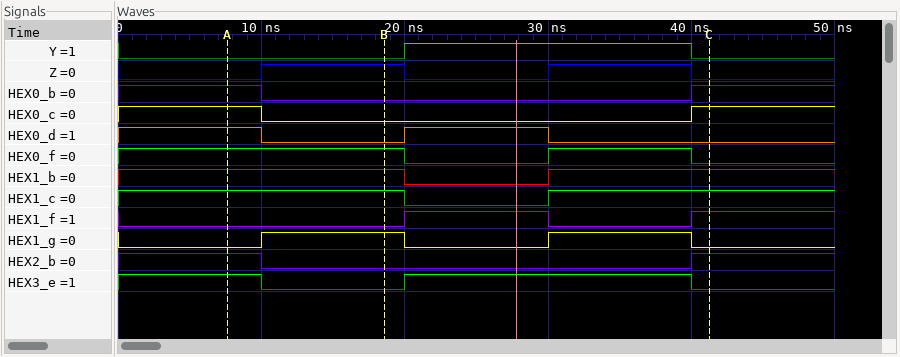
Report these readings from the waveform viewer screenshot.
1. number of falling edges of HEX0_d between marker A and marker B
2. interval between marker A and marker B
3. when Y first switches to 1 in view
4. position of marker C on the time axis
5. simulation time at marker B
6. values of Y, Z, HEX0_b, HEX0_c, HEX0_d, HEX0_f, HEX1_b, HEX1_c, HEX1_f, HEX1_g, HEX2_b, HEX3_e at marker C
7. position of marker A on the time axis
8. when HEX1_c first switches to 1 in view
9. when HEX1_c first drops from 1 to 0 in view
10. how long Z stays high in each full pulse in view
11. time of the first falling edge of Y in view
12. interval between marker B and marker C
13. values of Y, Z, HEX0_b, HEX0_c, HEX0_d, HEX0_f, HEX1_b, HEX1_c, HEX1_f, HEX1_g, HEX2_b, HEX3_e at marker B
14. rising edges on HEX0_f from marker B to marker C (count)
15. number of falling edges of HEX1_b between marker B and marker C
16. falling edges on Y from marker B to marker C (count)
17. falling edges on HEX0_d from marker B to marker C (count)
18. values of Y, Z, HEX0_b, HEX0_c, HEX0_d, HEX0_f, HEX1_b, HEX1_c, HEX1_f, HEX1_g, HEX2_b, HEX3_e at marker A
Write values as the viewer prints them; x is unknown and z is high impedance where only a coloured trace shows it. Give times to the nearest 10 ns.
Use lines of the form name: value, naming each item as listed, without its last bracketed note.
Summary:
number of falling edges of HEX0_d between marker A and marker B: 1
interval between marker A and marker B: 10 ns
when Y first switches to 1 in view: 20 ns
position of marker C on the time axis: 40 ns
simulation time at marker B: 20 ns
values of Y, Z, HEX0_b, HEX0_c, HEX0_d, HEX0_f, HEX1_b, HEX1_c, HEX1_f, HEX1_g, HEX2_b, HEX3_e at marker C: Y=0, Z=0, HEX0_b=1, HEX0_c=1, HEX0_d=0, HEX0_f=0, HEX1_b=1, HEX1_c=1, HEX1_f=1, HEX1_g=0, HEX2_b=1, HEX3_e=0
position of marker A on the time axis: 10 ns
when HEX1_c first switches to 1 in view: 30 ns
when HEX1_c first drops from 1 to 0 in view: 20 ns
how long Z stays high in each full pulse in view: 10 ns, 10 ns
time of the first falling edge of Y in view: 40 ns
interval between marker B and marker C: 20 ns
values of Y, Z, HEX0_b, HEX0_c, HEX0_d, HEX0_f, HEX1_b, HEX1_c, HEX1_f, HEX1_g, HEX2_b, HEX3_e at marker B: Y=0, Z=1, HEX0_b=0, HEX0_c=0, HEX0_d=0, HEX0_f=1, HEX1_b=1, HEX1_c=1, HEX1_f=0, HEX1_g=1, HEX2_b=0, HEX3_e=0
rising edges on HEX0_f from marker B to marker C: 1
number of falling edges of HEX1_b between marker B and marker C: 1
falling edges on Y from marker B to marker C: 1
falling edges on HEX0_d from marker B to marker C: 1
values of Y, Z, HEX0_b, HEX0_c, HEX0_d, HEX0_f, HEX1_b, HEX1_c, HEX1_f, HEX1_g, HEX2_b, HEX3_e at marker A: Y=0, Z=0, HEX0_b=1, HEX0_c=1, HEX0_d=1, HEX0_f=1, HEX1_b=1, HEX1_c=1, HEX1_f=0, HEX1_g=0, HEX2_b=1, HEX3_e=1
